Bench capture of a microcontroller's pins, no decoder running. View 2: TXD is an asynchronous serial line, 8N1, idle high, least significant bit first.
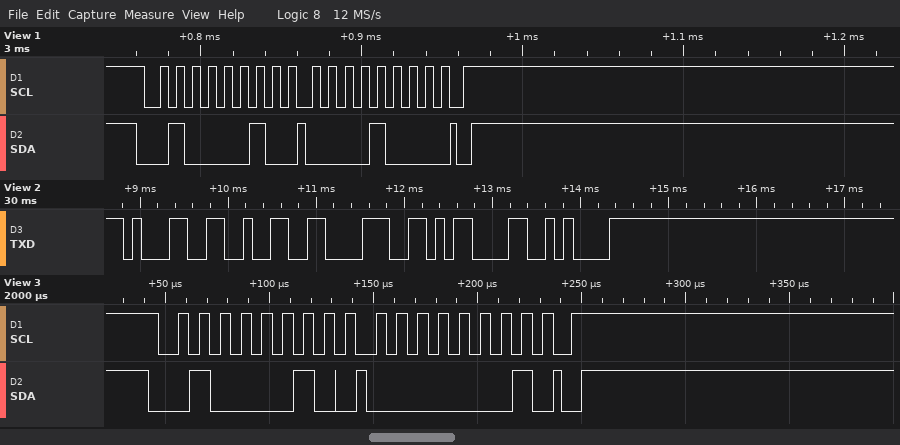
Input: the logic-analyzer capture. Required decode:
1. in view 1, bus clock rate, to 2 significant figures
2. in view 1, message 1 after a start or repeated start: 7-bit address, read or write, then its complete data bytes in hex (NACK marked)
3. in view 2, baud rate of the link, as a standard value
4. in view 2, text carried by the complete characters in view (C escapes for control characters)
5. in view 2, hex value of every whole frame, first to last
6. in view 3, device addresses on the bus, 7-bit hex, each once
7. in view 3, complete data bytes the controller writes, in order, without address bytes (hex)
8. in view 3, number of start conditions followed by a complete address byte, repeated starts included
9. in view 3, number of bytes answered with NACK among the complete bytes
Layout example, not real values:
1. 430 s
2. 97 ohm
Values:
1. 100 kHz
2. 0x21 write: 08
3. 9600 baud
4. "128\r\n"
5. 31 32 38 0D 0A
6. 0x21
7. 01
8. 1
9. 0
